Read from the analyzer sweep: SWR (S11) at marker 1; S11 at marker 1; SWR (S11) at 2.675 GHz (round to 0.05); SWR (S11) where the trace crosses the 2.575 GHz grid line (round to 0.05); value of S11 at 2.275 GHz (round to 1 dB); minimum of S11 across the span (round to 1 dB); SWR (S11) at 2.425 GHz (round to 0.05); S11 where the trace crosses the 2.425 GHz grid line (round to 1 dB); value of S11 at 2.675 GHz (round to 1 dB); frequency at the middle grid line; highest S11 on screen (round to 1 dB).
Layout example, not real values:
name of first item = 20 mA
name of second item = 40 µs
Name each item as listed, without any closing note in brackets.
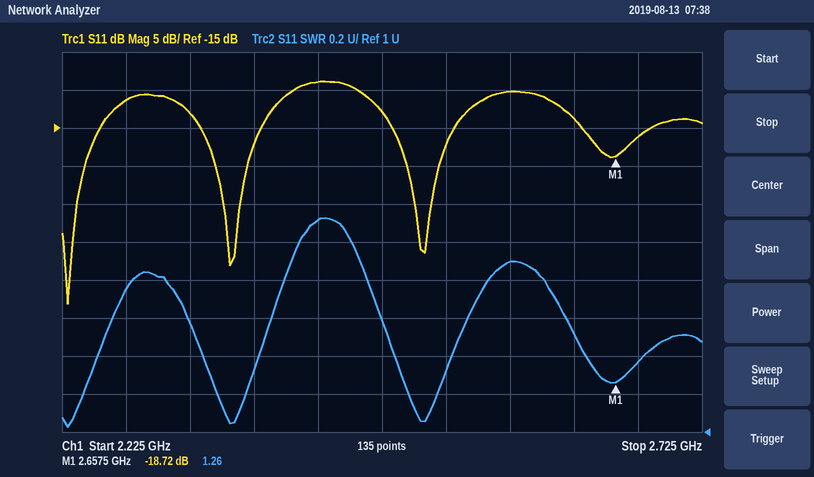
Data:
SWR (S11) at marker 1 = 1.26
S11 at marker 1 = -18.72 dB
SWR (S11) at 2.675 GHz = 1.35
SWR (S11) where the trace crosses the 2.575 GHz grid line = 1.90
value of S11 at 2.275 GHz = -11 dB
minimum of S11 across the span = -38 dB
SWR (S11) at 2.425 GHz = 2.10
S11 where the trace crosses the 2.425 GHz grid line = -9 dB
value of S11 at 2.675 GHz = -16 dB
frequency at the middle grid line = 2.475 GHz
highest S11 on screen = -9 dB
